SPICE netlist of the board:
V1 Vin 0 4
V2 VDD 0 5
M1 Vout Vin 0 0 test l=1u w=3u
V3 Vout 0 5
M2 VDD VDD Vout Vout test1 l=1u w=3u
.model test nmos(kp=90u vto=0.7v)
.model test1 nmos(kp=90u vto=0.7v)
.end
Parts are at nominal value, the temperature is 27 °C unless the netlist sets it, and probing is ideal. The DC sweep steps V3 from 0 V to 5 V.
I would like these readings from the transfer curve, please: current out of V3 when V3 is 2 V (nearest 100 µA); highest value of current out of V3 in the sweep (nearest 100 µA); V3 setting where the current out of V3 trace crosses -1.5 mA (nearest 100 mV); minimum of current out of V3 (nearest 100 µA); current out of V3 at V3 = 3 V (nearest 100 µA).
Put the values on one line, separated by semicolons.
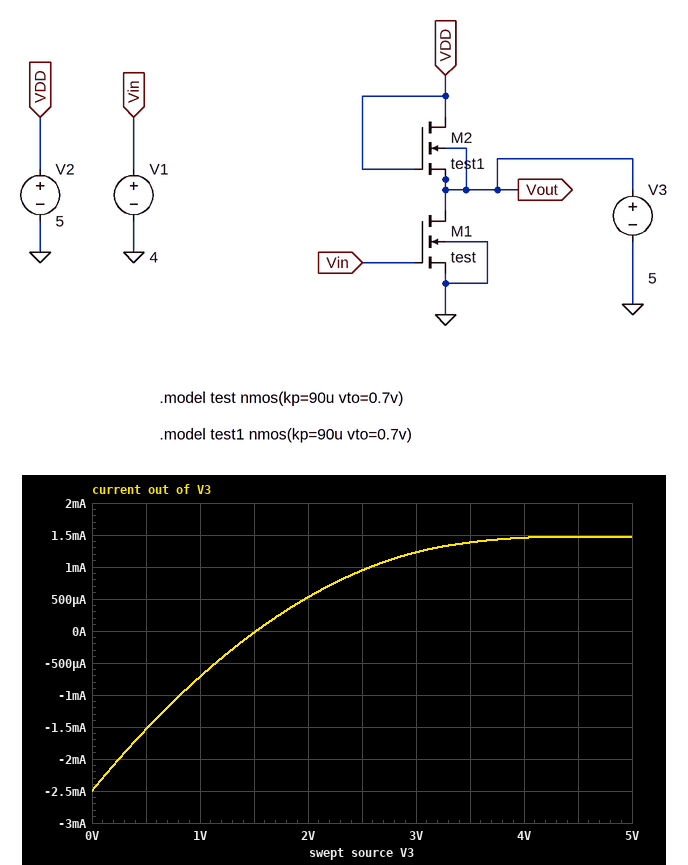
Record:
500 µA; 1.5 mA; 500 mV; -2.5 mA; 1.2 mA
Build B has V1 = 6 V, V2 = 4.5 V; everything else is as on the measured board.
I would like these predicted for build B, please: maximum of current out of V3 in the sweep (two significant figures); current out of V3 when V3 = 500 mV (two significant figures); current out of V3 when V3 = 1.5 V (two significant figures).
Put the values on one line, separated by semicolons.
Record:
3.8 mA; -790 µA; 1.1 mA
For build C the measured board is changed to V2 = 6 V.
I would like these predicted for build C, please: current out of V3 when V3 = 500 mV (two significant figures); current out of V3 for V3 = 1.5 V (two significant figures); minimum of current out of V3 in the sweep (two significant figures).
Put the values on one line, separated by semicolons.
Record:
-2.7 mA; -920 µA; -3.8 mA
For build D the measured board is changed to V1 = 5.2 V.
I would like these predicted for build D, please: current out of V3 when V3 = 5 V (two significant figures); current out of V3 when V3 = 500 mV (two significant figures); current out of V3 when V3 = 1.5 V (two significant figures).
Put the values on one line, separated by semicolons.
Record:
2.7 mA; -1.4 mA; 460 µA
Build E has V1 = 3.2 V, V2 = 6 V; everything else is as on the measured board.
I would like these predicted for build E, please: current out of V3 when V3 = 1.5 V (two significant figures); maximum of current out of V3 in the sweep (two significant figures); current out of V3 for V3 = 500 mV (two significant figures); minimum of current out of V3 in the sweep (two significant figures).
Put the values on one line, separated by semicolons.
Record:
-1.2 mA; 830 µA; -2.8 mA; -3.8 mA
